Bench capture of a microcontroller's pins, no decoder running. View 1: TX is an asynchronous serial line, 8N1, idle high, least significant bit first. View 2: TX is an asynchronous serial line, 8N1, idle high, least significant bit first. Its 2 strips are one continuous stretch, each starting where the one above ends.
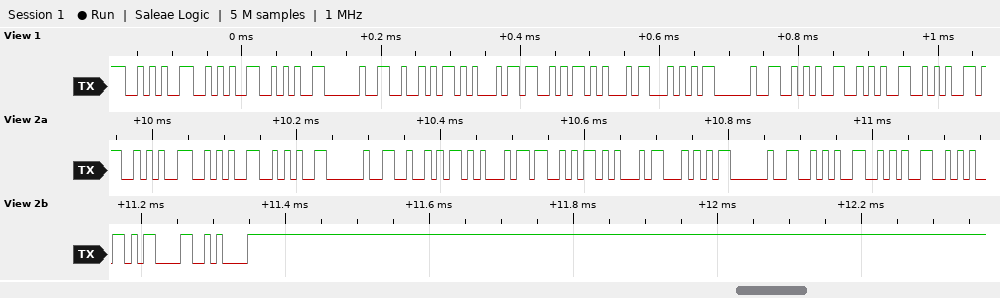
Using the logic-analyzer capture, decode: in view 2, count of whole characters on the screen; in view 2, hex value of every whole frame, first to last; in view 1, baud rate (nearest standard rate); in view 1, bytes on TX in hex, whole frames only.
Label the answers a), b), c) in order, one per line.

a) 15
b) 0x2A 0x2A 0x2A 0x20 0x52 0x45 0x53 0x45 0x54 0x20 0x2A 0x2A 0x2A 0x0D 0x0A
c) 115200 baud
d) 2A 2A 2A 20 52 45 53 45 54 20 2A 2A 2A
